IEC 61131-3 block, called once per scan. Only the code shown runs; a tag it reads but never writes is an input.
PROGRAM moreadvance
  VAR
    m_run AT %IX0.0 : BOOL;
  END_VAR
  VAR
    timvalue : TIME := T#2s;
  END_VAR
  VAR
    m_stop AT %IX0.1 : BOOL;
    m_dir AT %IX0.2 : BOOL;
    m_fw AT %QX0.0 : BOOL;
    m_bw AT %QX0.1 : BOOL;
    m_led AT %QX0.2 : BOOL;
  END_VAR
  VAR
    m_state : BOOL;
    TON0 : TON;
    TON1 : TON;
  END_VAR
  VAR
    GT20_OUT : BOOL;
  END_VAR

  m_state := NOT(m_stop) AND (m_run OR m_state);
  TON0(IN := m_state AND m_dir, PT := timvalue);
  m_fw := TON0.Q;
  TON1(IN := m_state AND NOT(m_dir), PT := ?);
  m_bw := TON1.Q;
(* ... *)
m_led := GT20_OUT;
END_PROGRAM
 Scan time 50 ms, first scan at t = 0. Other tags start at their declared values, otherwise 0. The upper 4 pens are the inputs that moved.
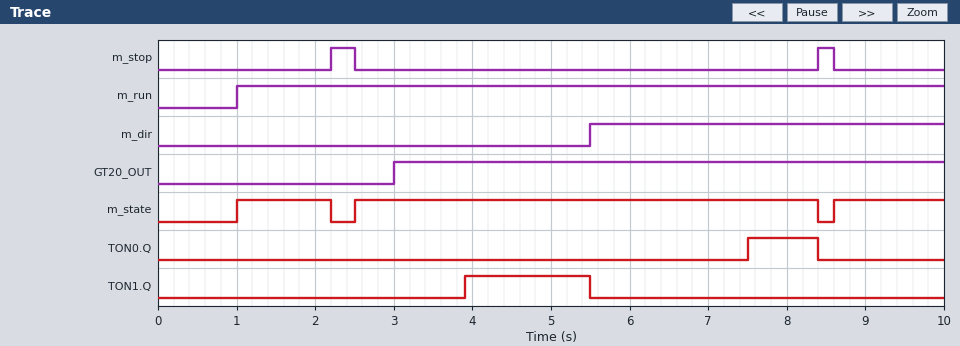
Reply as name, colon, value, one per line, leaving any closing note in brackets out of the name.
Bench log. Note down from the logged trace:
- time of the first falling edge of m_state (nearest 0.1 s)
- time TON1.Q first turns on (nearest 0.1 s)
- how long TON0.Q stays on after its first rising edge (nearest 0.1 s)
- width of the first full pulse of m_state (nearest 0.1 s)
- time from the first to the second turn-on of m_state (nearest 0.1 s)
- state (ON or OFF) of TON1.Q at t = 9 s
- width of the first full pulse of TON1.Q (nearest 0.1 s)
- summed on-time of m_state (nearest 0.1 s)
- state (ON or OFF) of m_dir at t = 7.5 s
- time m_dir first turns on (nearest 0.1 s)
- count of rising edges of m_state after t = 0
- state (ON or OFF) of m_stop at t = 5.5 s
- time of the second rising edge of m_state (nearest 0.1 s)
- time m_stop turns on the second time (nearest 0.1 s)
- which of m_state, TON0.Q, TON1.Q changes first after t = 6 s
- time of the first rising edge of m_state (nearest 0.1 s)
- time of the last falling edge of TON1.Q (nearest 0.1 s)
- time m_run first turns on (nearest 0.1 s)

time of the first falling edge of m_state: 2.2 s
time TON1.Q first turns on: 3.9 s
how long TON0.Q stays on after its first rising edge: 0.9 s
width of the first full pulse of m_state: 1.2 s
time from the first to the second turn-on of m_state: 1.5 s
state (ON or OFF) of TON1.Q at t = 9 s: OFF
width of the first full pulse of TON1.Q: 1.6 s
summed on-time of m_state: 8.5 s
state (ON or OFF) of m_dir at t = 7.5 s: ON
time m_dir first turns on: 5.5 s
count of rising edges of m_state after t = 0: 3
state (ON or OFF) of m_stop at t = 5.5 s: OFF
time of the second rising edge of m_state: 2.5 s
time m_stop turns on the second time: 8.4 s
which of m_state, TON0.Q, TON1.Q changes first after t = 6 s: TON0.Q
time of the first rising edge of m_state: 1.0 s
time of the last falling edge of TON1.Q: 5.5 s
time m_run first turns on: 1.0 s
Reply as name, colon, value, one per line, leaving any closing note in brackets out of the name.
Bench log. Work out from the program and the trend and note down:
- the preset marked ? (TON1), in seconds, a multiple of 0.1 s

the preset marked ? (TON1), in seconds, a multiple of 0.1 s: 1.4 s
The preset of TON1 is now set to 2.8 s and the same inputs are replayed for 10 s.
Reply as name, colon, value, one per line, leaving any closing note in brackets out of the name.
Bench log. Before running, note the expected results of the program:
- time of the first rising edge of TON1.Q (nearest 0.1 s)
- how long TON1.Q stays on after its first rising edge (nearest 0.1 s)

time of the first rising edge of TON1.Q: 5.3 s
how long TON1.Q stays on after its first rising edge: 0.2 s
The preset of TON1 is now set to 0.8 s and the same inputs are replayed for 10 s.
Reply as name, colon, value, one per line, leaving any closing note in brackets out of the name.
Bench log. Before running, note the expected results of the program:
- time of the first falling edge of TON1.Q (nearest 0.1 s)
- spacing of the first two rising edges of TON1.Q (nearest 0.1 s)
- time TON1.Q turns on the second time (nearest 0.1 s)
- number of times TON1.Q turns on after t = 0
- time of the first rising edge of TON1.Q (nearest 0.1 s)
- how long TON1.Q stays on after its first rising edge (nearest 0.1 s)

time of the first falling edge of TON1.Q: 2.2 s
spacing of the first two rising edges of TON1.Q: 1.5 s
time TON1.Q turns on the second time: 3.3 s
number of times TON1.Q turns on after t = 0: 2
time of the first rising edge of TON1.Q: 1.8 s
how long TON1.Q stays on after its first rising edge: 0.4 s
